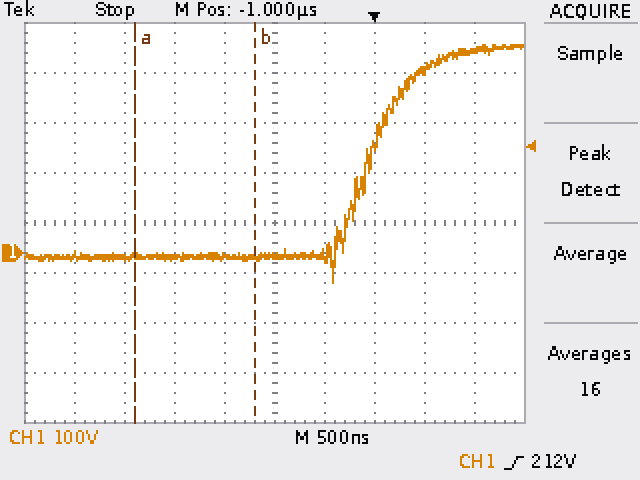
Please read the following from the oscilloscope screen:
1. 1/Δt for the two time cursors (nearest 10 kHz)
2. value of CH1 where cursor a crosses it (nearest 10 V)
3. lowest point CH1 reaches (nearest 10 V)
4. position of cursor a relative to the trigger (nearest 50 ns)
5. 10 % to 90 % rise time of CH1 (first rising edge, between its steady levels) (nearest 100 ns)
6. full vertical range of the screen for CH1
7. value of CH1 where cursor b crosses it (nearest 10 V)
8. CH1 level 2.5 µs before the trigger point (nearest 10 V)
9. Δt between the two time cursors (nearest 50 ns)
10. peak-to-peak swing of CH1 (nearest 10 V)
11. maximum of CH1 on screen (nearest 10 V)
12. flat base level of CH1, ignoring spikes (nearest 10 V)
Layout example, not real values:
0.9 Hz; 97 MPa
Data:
830 kHz; -10 V; -60 V; -2.40 µs; 800 ns; 800 V; -10 V; -10 V; 1.20 µs; 480 V; 420 V; -10 V
